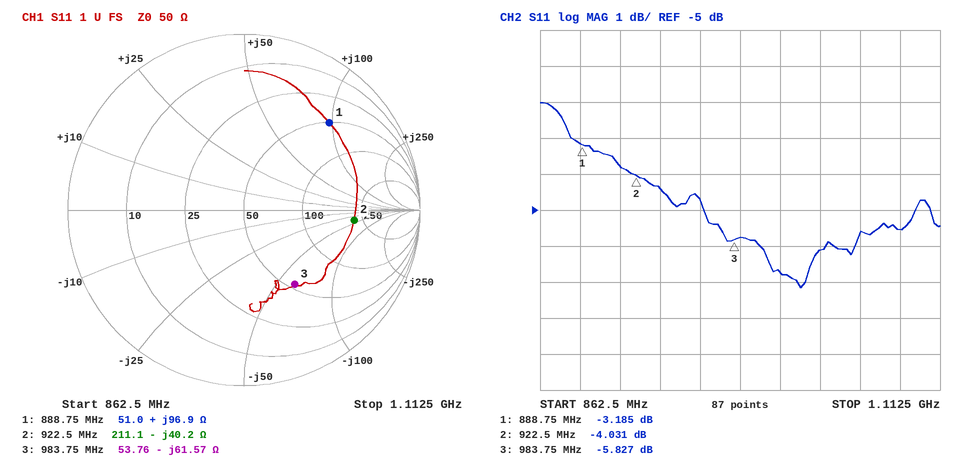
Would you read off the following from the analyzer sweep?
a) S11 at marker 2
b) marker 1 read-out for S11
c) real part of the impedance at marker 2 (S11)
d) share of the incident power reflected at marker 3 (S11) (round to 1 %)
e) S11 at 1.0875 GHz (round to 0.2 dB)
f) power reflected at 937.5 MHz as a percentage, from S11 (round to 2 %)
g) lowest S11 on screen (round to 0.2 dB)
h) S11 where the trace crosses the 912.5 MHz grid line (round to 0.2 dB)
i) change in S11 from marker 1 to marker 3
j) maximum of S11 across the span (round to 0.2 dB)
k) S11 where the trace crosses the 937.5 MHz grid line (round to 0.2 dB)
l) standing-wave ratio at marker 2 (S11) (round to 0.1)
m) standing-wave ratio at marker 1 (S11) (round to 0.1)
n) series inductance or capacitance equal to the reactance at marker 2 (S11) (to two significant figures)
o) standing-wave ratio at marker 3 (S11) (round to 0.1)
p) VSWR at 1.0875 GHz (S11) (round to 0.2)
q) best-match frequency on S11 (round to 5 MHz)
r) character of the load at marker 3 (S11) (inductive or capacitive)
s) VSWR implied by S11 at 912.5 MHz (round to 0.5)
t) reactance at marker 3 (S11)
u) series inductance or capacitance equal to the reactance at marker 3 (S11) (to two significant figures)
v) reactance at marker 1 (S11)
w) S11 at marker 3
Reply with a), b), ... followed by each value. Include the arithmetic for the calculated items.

a) -4.031 dB
b) -3.185 dB
c) 211.1 Ω
d) 10^(-5.827/10) ≈ 26 %
e) -5.6 dB
f) 10^(-4.4/10) ≈ 36 %
g) -7.2 dB
h) -3.8 dB
i) -5.827 − (-3.185) = -2.642 dB
j) -2.0 dB
k) -4.4 dB
l) 4.4
m) 5.5
n) C = 1/(2π × 922.5 MHz × 40.2 Ω) ≈ 4.3 pF
o) 3.1
p) |Γ| = 10^(-5.6/20) = 0.5248; VSWR = (1 + 0.5248)/(1 − 0.5248) ≈ 3.2
q) 1.025 GHz
r) capacitive
s) |Γ| = 10^(-3.8/20) = 0.6457; VSWR = (1 + 0.6457)/(1 − 0.6457) ≈ 4.64, so 4.5 to the nearest 0.5
t) -61.57 Ω
u) C = 1/(2π × 983.75 MHz × 61.57 Ω) ≈ 2.6 pF
v) +96.9 Ω
w) -5.827 dB
